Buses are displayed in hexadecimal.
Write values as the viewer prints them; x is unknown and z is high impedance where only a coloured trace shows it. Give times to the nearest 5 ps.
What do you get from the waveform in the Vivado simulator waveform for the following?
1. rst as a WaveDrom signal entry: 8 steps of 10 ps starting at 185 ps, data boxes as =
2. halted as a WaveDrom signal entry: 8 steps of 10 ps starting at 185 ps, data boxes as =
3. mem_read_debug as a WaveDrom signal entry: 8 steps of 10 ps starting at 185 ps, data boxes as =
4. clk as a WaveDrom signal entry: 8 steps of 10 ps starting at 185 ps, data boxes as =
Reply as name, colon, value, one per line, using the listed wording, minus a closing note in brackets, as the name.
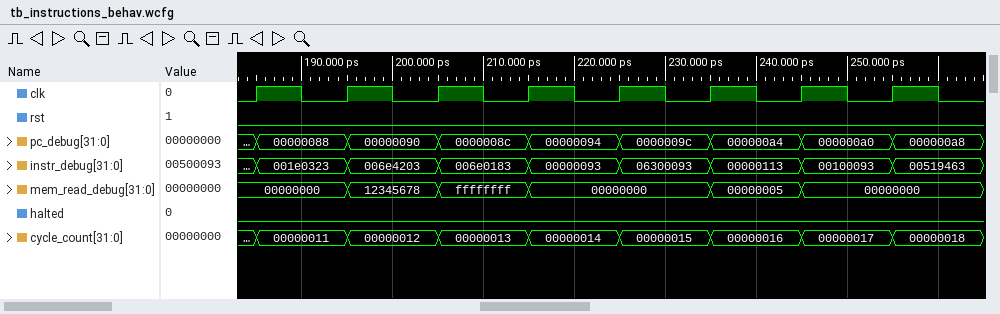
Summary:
rst as a WaveDrom signal entry: 8 steps of 10 ps starting at 185 ps, data boxes as =: {name: 'rst', wave: '0.......'}
halted as a WaveDrom signal entry: 8 steps of 10 ps starting at 185 ps, data boxes as =: {name: 'halted', wave: '0.......'}
mem_read_debug as a WaveDrom signal entry: 8 steps of 10 ps starting at 185 ps, data boxes as =: {name: 'mem_read_debug', wave: '====.==.', data: '00000000 12345678 ffffffff 00000000 00000005 00000000'}
clk as a WaveDrom signal entry: 8 steps of 10 ps starting at 185 ps, data boxes as =: {name: 'clk', wave: 'p.......'}
